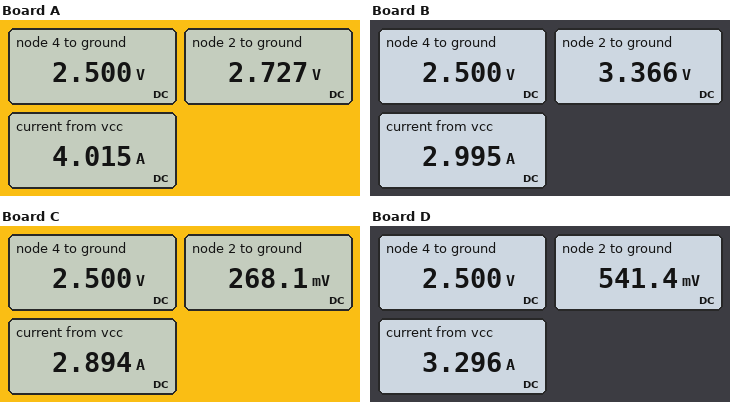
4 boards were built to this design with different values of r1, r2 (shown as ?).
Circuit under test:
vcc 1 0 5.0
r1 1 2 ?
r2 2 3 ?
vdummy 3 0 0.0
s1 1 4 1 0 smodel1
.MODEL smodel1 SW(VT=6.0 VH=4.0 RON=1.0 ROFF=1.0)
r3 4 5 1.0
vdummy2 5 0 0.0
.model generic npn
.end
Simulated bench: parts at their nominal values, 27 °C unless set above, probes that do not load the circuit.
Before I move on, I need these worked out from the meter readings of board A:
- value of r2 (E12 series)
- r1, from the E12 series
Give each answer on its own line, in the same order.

1.8 Ω
1.5 Ω
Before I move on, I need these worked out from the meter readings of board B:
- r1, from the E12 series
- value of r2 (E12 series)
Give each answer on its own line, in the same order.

3.3 Ω
6.8 Ω
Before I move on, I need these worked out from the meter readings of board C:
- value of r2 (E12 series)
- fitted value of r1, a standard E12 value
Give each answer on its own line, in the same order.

0.68 Ω
12 Ω
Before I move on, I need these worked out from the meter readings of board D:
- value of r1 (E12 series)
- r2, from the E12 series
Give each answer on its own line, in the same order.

5.6 Ω
0.68 Ω
